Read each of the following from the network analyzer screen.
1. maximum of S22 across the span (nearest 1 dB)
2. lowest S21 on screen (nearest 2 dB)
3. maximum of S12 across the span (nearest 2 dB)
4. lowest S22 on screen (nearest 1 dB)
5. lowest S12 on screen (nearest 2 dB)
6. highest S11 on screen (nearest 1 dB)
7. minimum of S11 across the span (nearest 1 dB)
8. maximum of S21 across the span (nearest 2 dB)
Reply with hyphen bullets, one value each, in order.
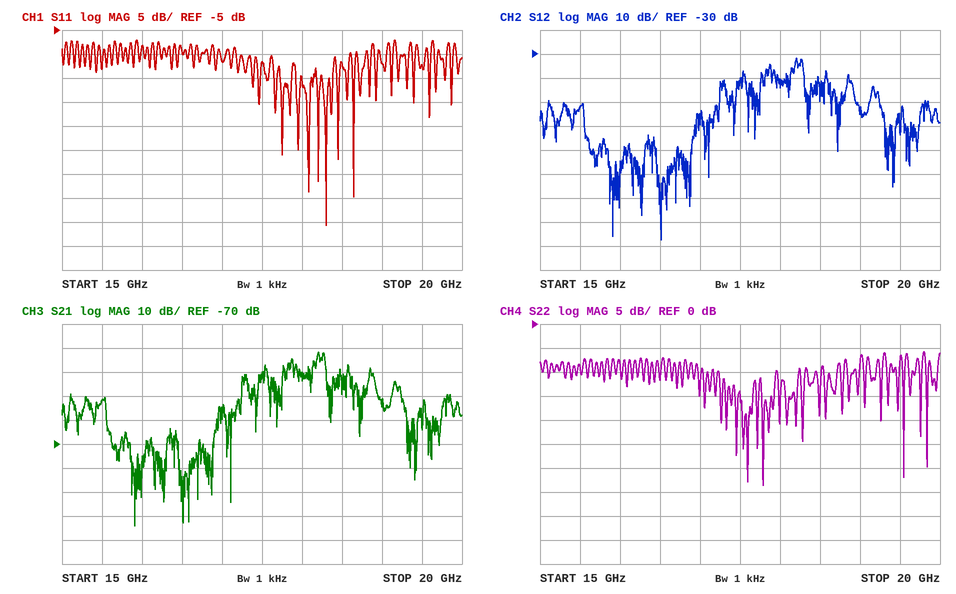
- -6 dB
- -104 dB
- -32 dB
- -34 dB
- -108 dB
- -7 dB
- -46 dB
- -32 dB
